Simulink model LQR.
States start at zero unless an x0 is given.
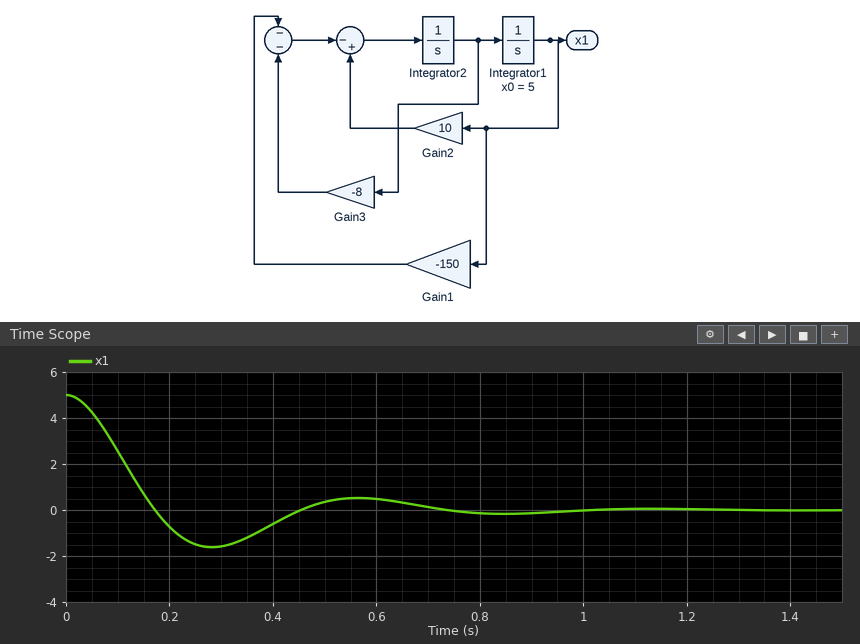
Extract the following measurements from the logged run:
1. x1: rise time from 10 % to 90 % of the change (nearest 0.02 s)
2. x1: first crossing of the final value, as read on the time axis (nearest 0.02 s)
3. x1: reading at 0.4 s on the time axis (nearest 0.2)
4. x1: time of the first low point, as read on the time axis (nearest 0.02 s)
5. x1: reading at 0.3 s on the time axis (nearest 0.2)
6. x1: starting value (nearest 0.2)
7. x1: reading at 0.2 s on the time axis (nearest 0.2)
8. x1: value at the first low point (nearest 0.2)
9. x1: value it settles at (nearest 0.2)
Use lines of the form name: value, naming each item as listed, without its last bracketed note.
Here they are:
x1: rise time from 10 % to 90 % of the change: 0.12 s
x1: first crossing of the final value, as read on the time axis: 0.18 s
x1: reading at 0.4 s on the time axis: -0.6
x1: time of the first low point, as read on the time axis: 0.28 s
x1: reading at 0.3 s on the time axis: -1.6
x1: starting value: 5.0
x1: reading at 0.2 s on the time axis: -0.8
x1: value at the first low point: -1.6
x1: value it settles at: 0.0
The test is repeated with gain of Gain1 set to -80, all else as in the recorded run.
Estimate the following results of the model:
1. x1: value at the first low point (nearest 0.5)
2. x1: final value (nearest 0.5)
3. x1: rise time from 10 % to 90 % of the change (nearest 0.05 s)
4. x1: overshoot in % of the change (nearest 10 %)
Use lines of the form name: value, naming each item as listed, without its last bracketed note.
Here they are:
x1: value at the first low point: -1.0
x1: final value: 0.0
x1: rise time from 10 % to 90 % of the change: 0.20 s
x1: overshoot in % of the change: 20 %
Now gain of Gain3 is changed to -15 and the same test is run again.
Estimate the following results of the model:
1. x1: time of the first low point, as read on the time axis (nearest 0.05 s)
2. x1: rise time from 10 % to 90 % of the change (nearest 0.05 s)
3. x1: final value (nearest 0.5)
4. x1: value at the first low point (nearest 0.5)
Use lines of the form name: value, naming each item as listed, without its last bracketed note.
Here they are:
x1: time of the first low point, as read on the time axis: 0.35 s
x1: rise time from 10 % to 90 % of the change: 0.15 s
x1: final value: 0.0
x1: value at the first low point: -0.5
